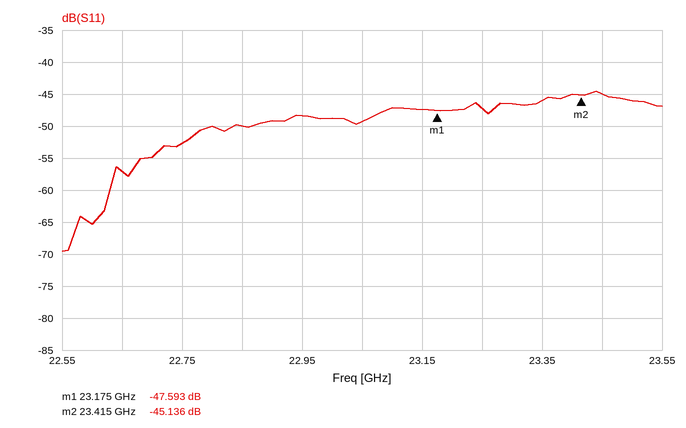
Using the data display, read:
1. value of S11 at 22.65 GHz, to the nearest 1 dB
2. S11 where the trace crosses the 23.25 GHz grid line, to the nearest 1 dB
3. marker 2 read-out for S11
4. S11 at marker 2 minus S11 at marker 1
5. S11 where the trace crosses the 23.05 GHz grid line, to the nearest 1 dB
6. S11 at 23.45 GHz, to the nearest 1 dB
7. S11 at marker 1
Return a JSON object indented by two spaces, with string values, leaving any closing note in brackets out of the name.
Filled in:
{
  "value of S11 at 22.65 GHz, to the nearest 1 dB": "-57 dB",
  "S11 where the trace crosses the 23.25 GHz grid line, to the nearest 1 dB": "-47 dB",
  "marker 2 read-out for S11": "-45.136 dB",
  "S11 at marker 2 minus S11 at marker 1": "2.457 dB",
  "S11 where the trace crosses the 23.05 GHz grid line, to the nearest 1 dB": "-49 dB",
  "S11 at 23.45 GHz, to the nearest 1 dB": "-45 dB",
  "S11 at marker 1": "-47.593 dB"
}
